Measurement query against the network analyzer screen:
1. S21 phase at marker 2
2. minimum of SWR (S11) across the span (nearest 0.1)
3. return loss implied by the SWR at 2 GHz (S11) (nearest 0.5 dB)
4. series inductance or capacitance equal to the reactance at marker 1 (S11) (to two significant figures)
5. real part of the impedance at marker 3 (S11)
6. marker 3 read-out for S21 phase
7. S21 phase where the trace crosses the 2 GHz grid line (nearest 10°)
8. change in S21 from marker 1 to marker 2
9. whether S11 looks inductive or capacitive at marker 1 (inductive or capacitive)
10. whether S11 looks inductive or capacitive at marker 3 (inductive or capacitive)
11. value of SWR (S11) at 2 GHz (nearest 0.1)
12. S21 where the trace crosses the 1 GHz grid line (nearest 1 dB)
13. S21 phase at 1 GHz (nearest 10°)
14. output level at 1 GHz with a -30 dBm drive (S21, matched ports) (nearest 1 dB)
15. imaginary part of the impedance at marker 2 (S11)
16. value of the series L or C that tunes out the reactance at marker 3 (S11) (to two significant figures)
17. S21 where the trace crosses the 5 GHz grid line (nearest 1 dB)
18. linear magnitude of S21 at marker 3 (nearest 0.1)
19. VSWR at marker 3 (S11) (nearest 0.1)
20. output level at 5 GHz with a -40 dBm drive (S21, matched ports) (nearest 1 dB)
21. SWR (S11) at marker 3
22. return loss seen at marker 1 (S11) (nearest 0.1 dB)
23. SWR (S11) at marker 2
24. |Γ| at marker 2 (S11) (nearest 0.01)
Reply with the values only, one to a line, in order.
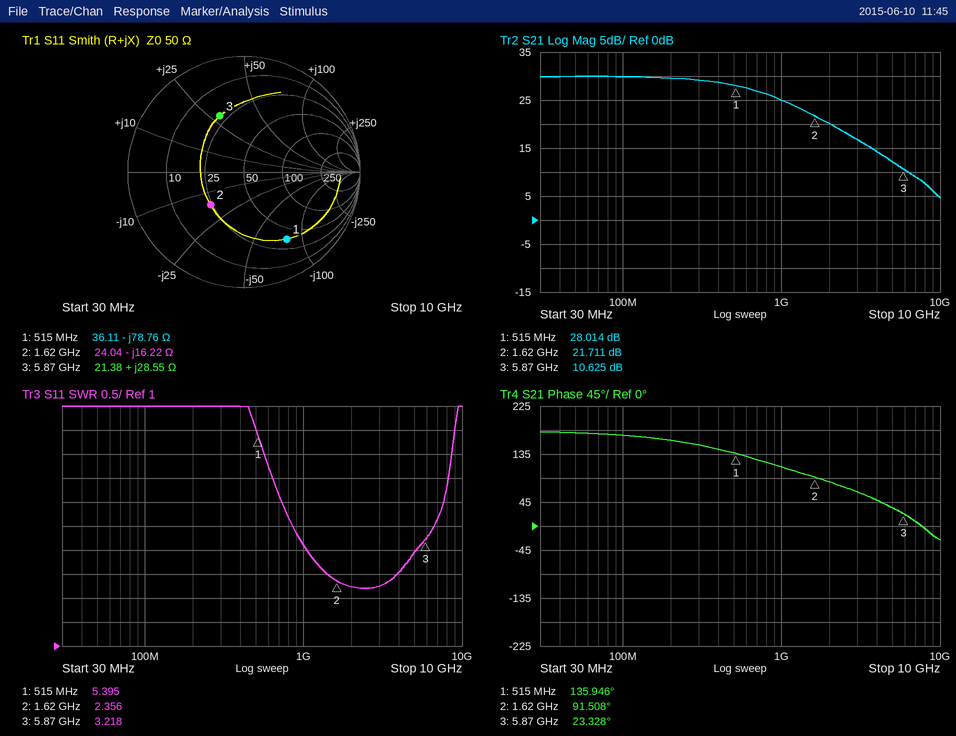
91.508°
2.2
8.5 dB
3.9 pF
21.38 Ω
23.328°
80°
-6.303 dB
capacitive
inductive
2.2
25 dB
110°
-5 dBm
-16.22 Ω
950 fF
12 dB
3.4
3.2
-28 dBm
3.218
3.3 dB
2.356
0.40
